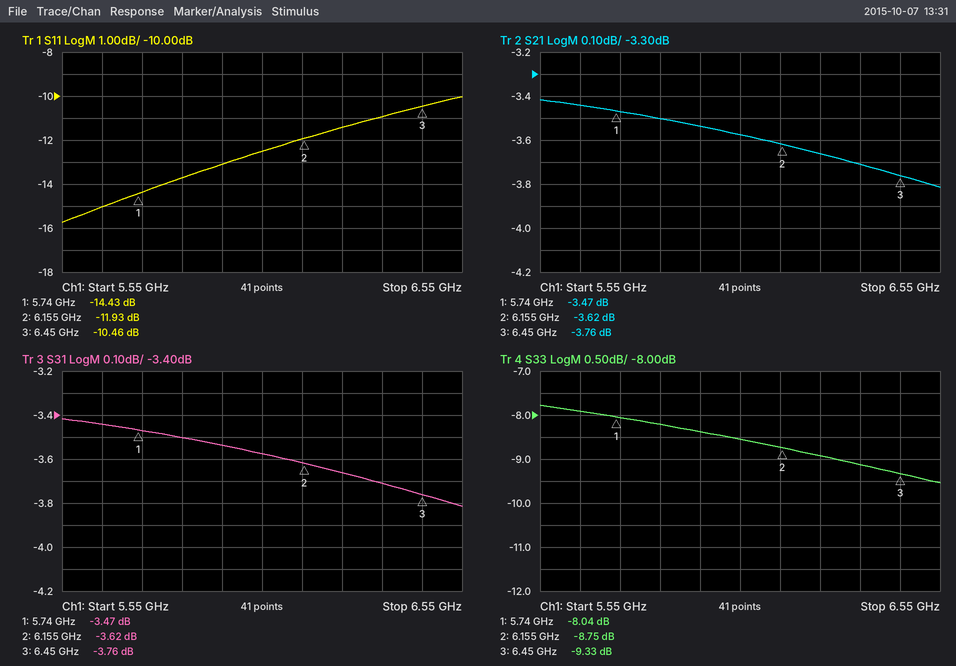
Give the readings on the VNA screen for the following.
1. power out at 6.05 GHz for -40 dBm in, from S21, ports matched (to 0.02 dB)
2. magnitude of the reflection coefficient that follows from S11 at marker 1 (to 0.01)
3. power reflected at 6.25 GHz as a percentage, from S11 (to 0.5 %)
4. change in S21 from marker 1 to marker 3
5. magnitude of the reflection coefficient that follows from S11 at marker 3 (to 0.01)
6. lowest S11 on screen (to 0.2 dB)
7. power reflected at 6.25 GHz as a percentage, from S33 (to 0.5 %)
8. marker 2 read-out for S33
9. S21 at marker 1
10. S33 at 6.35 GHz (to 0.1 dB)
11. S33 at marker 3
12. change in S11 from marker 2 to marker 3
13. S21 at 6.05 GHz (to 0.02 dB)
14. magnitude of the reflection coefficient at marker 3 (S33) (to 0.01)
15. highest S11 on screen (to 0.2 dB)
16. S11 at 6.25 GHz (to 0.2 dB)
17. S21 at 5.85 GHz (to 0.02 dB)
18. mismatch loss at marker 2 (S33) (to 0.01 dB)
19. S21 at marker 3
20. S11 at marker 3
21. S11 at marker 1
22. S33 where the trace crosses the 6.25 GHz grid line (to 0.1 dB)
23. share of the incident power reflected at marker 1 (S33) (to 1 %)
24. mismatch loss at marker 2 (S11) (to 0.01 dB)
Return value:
-43.58 dBm
0.19
7.0 %
-0.29 dB
0.30
-15.8 dB
13.0 %
-8.75 dB
-3.47 dB
-9.1 dB
-9.33 dB
1.47 dB
-3.58 dB
0.34
-10.0 dB
-11.4 dB
-3.50 dB
0.62 dB
-3.76 dB
-10.46 dB
-14.43 dB
-8.9 dB
16 %
0.29 dB
